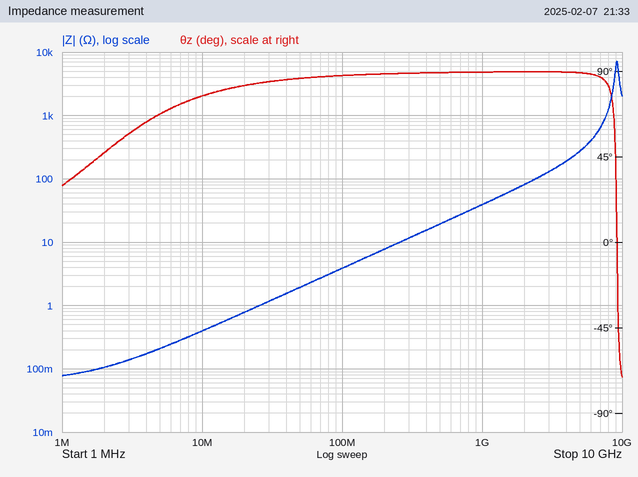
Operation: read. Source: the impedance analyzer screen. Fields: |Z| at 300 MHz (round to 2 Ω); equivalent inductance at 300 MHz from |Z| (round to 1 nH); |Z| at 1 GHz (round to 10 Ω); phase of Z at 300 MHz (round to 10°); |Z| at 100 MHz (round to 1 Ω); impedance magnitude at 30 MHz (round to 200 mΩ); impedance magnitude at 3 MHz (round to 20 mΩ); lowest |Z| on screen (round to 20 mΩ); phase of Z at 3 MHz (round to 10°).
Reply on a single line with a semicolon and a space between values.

12 Ω; 6 nH; 40 Ω; 90°; 4 Ω; 1.2 Ω; 140 mΩ; 80 mΩ; 60°
